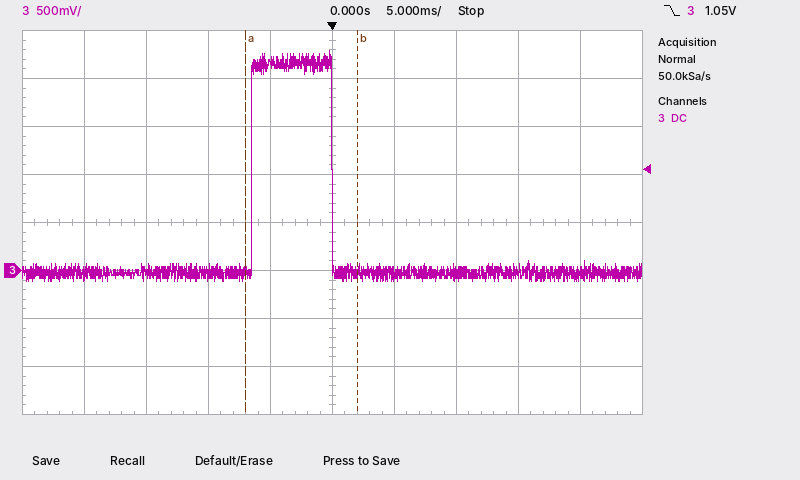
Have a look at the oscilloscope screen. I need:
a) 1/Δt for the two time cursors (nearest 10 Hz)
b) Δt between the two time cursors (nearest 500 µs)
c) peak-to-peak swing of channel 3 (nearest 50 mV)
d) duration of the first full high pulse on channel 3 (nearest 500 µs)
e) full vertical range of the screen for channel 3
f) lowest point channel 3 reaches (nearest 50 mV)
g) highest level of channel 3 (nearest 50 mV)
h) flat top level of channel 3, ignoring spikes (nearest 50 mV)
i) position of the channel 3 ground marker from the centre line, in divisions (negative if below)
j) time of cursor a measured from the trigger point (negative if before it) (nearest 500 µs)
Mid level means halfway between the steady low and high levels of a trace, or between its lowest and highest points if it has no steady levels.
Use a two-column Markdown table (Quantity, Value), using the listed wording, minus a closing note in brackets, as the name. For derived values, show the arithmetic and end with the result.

| Quantity | Value |
|---|---|
| 1/Δt for the two time cursors | 1 / 9.0 ms ≈ 110 Hz |
| Δt between the two time cursors | 9.0 ms |
| peak-to-peak swing of channel 3 | 2.30 V − (-100 mV) = 2.40 V |
| duration of the first full high pulse on channel 3 | 6.5 ms |
| full vertical range of the screen for channel 3 | 4 V |
| lowest point channel 3 reaches | -100 mV |
| highest level of channel 3 | 2.30 V |
| flat top level of channel 3, ignoring spikes | 2.15 V |
| position of the channel 3 ground marker from the centre line, in divisions | -1.0 div |
| time of cursor a measured from the trigger point (negative if before it) | -7.0 ms |
